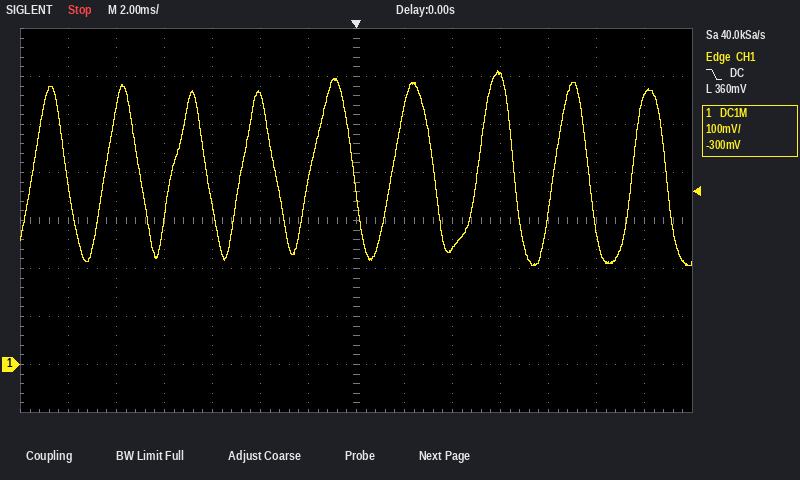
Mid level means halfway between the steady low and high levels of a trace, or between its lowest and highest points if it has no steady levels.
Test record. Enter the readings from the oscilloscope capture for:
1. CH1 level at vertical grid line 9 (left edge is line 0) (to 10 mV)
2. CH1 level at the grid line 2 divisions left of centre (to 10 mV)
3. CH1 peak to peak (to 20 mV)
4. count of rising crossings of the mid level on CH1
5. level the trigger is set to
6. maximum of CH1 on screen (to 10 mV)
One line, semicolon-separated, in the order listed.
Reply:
240 mV; 560 mV; 400 mV; 9; 360 mV; 610 mV
